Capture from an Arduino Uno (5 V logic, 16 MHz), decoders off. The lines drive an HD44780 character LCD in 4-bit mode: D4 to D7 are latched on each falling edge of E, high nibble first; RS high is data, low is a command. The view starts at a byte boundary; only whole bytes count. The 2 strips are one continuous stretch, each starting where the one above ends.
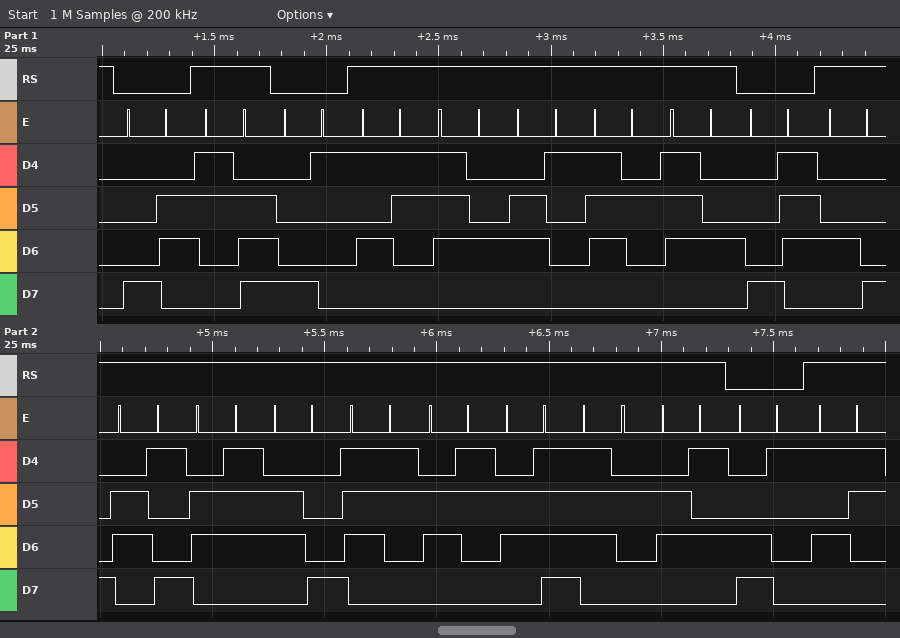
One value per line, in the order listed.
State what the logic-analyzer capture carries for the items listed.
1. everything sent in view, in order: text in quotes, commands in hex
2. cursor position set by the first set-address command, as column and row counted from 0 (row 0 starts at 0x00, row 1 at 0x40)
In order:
0x86 ">" 0x81 "Start" 0x87 "Highscore" 0xC1 "S"
column 6, row 0
